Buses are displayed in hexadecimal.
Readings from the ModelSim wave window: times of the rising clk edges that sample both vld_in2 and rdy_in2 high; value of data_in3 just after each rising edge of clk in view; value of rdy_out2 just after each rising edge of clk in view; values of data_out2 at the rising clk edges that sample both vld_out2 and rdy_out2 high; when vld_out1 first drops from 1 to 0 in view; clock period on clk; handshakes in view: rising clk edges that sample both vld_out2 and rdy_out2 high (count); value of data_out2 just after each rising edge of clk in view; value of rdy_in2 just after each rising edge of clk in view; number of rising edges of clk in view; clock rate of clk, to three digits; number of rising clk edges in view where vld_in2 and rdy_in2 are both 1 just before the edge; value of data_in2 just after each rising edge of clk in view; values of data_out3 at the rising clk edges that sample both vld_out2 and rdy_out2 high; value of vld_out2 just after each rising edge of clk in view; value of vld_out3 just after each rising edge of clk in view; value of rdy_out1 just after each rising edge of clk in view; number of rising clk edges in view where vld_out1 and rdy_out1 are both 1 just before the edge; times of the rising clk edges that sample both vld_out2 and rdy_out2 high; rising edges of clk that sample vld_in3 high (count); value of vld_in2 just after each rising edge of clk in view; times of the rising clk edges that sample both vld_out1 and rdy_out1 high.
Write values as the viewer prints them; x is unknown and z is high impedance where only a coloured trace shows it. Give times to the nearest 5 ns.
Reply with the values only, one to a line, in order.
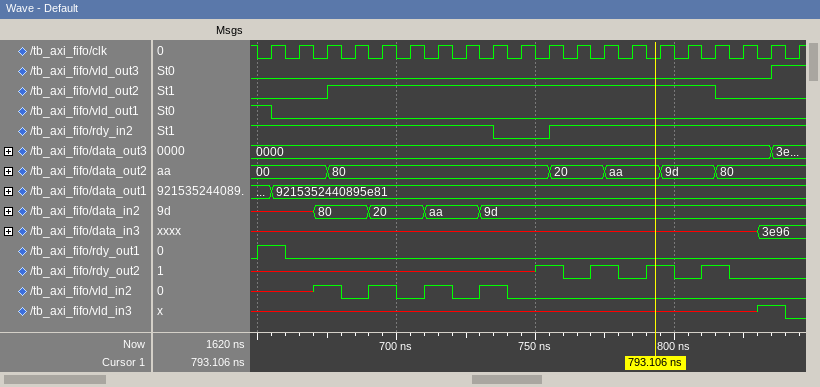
675 ns, 695 ns, 715 ns, 735 ns
x, x, x, x, x, x, x, x, x, x, x, x, x, x, x, x, x, x, 3e96, 3e96
x x x x x x x x x x 1 0 1 0 1 0 1 0 0 0
80, 20, aa, 9d
655 ns
10 ns
4
00, 00, 80, 80, 80, 80, 80, 80, 80, 80, 20, 20, aa, aa, 9d, 9d, 80, 80, 80, 80
1 1 1 1 1 1 1 1 0 0 1 1 1 1 1 1 1 1 1 1
20
100 MHz
4
x, x, 80, 80, 20, 20, aa, aa, 9d, 9d, 9d, 9d, 9d, 9d, 9d, 9d, 9d, 9d, 9d, 9d
0000, 0000, 0000, 0000
0 0 1 1 1 1 1 1 1 1 1 1 1 1 1 1 0 0 0 0
0 0 0 0 0 0 0 0 0 0 0 0 0 0 0 0 0 0 1 1
1 0 0 0 0 0 0 0 0 0 0 0 0 0 0 0 0 0 0 0
1
755 ns, 775 ns, 795 ns, 815 ns
1
x x 1 0 1 0 1 0 1 0 0 0 0 0 0 0 0 0 0 0
655 ns
